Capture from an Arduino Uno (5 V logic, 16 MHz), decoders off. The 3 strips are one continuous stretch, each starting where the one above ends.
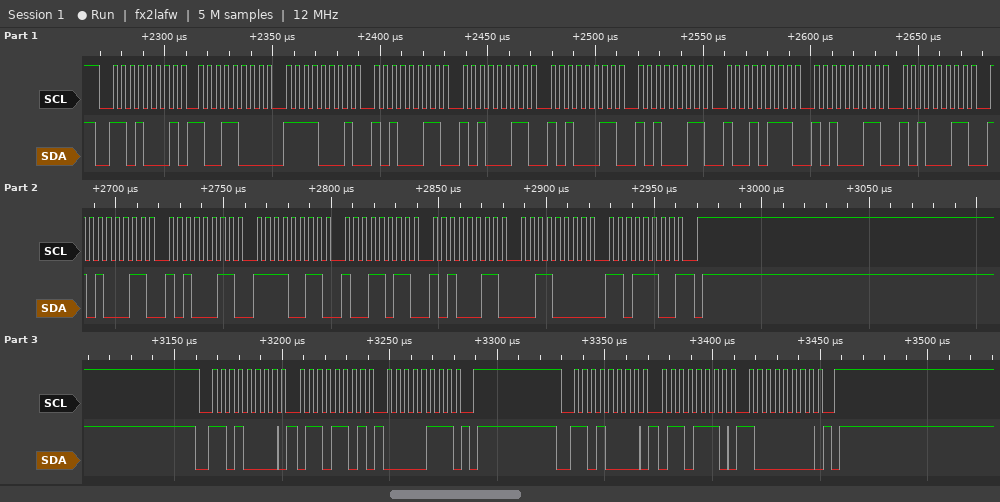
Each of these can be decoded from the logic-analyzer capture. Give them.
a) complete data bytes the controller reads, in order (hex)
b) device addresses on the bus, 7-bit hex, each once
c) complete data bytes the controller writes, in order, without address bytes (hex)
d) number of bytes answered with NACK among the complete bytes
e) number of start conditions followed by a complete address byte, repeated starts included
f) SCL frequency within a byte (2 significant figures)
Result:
98 F1 A3 A3 A3 A3 97 A3 A3 A3 A3 F3 9B A3 30 DC
0x68
6D 07 6E 80
1
3
250 kHz
